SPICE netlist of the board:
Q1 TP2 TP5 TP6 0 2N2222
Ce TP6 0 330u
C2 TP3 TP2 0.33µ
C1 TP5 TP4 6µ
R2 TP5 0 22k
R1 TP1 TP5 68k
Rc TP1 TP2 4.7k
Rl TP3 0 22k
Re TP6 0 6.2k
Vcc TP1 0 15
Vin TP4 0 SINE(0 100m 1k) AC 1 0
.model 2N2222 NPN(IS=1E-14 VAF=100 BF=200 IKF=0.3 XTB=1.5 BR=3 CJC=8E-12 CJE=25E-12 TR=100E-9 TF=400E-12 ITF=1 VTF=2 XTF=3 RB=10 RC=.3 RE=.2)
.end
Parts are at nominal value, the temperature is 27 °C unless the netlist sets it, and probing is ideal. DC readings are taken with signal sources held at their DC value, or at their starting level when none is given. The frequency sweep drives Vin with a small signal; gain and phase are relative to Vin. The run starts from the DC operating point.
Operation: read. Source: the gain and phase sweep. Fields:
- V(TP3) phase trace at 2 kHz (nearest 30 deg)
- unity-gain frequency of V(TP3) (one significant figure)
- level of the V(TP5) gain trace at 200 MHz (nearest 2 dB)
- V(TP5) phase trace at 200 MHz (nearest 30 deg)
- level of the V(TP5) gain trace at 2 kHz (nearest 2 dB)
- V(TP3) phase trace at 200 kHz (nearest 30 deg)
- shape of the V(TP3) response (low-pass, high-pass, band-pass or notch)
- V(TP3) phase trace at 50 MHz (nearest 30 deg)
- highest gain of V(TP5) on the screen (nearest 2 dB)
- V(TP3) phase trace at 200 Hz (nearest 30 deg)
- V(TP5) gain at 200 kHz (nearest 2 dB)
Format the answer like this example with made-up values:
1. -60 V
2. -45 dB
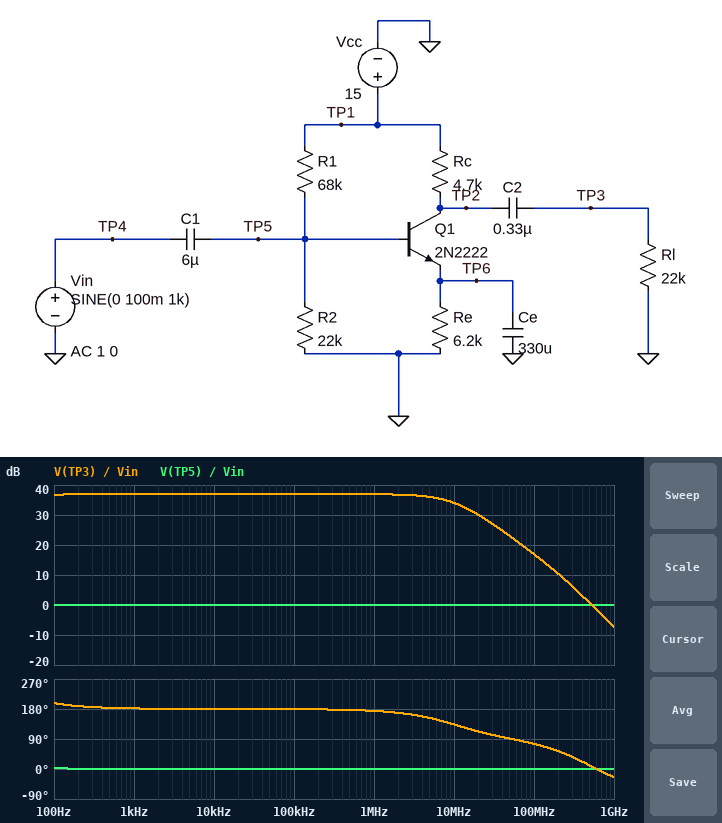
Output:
1. 180 deg
2. 500 MHz
3. 0 dB
4. 0 deg
5. 0 dB
6. 180 deg
7. low-pass
8. 90 deg
9. 0 dB
10. 180 deg
11. 0 dB
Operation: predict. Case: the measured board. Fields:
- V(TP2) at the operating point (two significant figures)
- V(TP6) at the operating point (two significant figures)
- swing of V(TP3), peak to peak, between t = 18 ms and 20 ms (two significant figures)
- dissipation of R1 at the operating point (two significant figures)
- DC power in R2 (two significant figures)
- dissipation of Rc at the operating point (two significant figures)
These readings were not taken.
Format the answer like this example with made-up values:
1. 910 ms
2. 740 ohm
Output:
1. 13 V
2. 3.0 V
3. 11 V
4. 1.9 mW
5. 600 µW
6. 1.1 mW
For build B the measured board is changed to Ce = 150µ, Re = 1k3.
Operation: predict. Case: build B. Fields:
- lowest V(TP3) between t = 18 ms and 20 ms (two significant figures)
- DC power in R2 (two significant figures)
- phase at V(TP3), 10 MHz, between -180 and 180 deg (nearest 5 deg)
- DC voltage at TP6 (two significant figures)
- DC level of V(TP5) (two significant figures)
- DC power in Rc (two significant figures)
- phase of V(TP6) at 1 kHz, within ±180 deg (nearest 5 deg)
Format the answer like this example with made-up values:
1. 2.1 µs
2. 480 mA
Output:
1. -7.4 V
2. 550 µW
3. 110 deg
4. 2.8 V
5. 3.5 V
6. 22 mW
7. -85 deg
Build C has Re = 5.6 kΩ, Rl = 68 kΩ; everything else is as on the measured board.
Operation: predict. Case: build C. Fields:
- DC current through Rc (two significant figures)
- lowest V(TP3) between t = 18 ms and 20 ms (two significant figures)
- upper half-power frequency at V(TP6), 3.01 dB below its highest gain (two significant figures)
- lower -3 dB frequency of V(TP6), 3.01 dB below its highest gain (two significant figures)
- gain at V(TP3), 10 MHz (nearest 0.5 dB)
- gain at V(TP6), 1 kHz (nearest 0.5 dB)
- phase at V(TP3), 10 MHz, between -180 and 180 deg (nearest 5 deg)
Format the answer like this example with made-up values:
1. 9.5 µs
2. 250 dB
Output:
1. 530 µA
2. -9.1 V
3. 15 Hz
4. 1.1 Hz
5. 35.5 dB
6. -40.5 dB
7. 130 deg
